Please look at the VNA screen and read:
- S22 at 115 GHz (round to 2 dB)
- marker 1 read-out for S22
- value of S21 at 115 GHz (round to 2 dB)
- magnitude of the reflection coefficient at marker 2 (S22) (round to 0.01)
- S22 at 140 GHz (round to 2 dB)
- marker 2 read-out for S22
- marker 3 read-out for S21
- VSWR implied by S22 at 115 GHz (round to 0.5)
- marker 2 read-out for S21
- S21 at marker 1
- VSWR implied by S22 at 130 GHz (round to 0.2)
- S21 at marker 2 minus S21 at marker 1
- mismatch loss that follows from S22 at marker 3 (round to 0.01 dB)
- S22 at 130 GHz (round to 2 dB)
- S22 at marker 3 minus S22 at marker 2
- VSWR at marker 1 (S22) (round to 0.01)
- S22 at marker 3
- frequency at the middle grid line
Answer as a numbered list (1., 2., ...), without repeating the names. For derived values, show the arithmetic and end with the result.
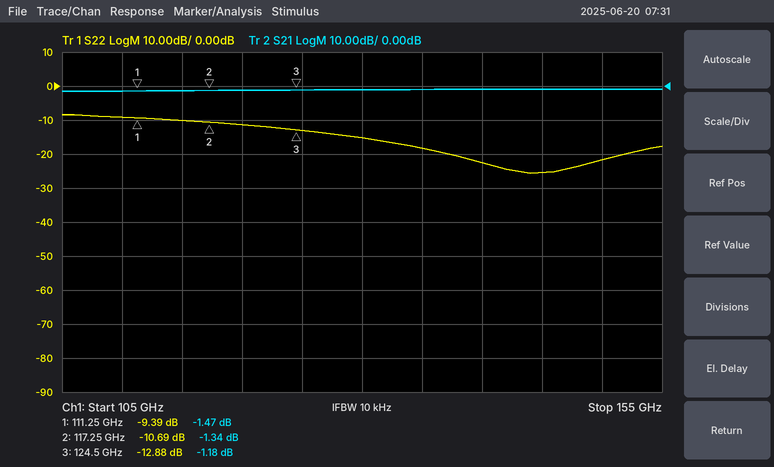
1. -10 dB
2. -9.39 dB
3. -2 dB
4. 10^(-10.69/20) ≈ 0.29
5. -22 dB
6. -10.69 dB
7. -1.18 dB
8. |Γ| = 10^(-10/20) = 0.3162; VSWR = (1 + 0.3162)/(1 − 0.3162) ≈ 1.92, so 2.0 to the nearest 0.5
9. -1.34 dB
10. -1.47 dB
11. |Γ| = 10^(-16/20) = 0.1585; VSWR = (1 + 0.1585)/(1 − 0.1585) ≈ 1.4
12. -1.34 − (-1.47) = 0.13 dB
13. −10 log10(1 − 10^(-12.88/10)) ≈ 0.23 dB
14. -16 dB
15. -12.88 − (-10.69) = -2.19 dB
16. (1 + 0.3392)/(1 − 0.3392) ≈ 2.03
17. -12.88 dB
18. 130 GHz
